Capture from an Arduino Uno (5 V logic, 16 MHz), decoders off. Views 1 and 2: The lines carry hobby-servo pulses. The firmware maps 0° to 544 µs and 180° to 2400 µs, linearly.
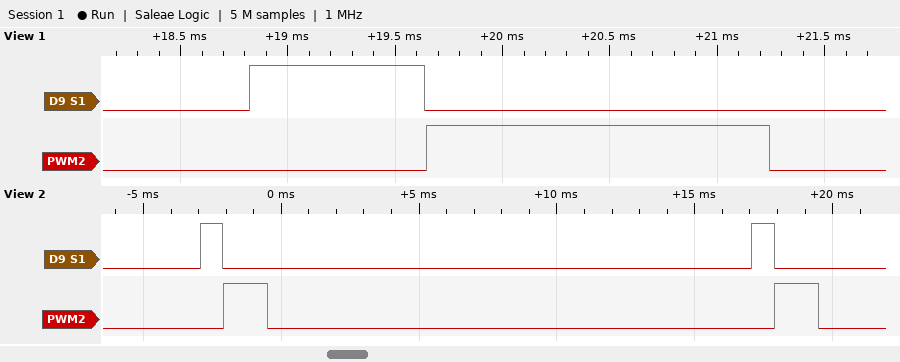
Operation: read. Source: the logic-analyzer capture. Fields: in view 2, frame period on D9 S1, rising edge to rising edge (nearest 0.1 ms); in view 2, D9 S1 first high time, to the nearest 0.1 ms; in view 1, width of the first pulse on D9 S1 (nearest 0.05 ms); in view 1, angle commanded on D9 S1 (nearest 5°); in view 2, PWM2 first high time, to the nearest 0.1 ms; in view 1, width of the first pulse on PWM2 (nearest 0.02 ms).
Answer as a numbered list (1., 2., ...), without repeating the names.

1. 20.0 ms
2. 0.8 ms
3. 0.80 ms
4. 25°
5. 1.6 ms
6. 1.60 ms
